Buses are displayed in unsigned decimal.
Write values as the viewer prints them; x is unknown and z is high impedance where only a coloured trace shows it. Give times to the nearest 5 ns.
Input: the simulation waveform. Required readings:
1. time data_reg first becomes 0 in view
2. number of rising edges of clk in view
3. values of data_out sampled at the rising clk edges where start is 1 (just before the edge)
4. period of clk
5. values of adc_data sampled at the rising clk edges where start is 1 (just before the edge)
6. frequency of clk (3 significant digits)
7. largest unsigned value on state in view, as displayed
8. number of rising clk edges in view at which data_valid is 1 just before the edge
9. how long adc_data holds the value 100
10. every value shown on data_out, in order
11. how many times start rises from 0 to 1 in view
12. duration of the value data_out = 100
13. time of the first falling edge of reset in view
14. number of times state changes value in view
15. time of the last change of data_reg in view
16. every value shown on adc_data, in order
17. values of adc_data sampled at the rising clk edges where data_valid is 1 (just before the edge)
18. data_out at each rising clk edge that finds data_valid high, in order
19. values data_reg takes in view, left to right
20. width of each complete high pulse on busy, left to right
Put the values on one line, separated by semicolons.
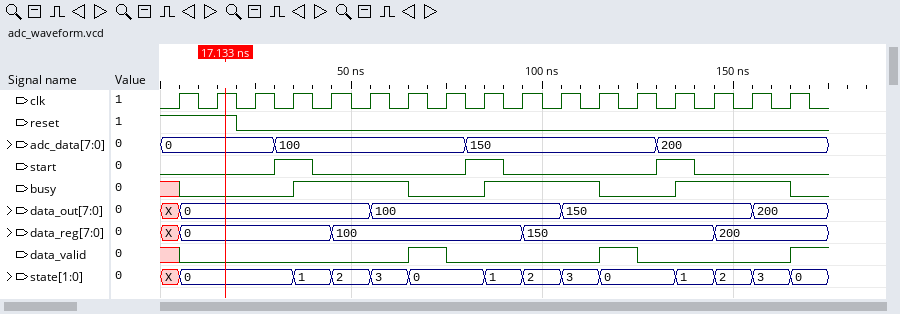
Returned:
5 ns; 17; 0, 100, 150; 10 ns; 100, 150, 200; 100 MHz; 3; 2; 50 ns; X, 0, 100, 150, 200; 3; 50 ns; 20 ns; 13; 145 ns; 0, 100, 150, 200; 100, 150; 100, 150; X, 0, 100, 150, 200; 30 ns, 30 ns, 30 ns
